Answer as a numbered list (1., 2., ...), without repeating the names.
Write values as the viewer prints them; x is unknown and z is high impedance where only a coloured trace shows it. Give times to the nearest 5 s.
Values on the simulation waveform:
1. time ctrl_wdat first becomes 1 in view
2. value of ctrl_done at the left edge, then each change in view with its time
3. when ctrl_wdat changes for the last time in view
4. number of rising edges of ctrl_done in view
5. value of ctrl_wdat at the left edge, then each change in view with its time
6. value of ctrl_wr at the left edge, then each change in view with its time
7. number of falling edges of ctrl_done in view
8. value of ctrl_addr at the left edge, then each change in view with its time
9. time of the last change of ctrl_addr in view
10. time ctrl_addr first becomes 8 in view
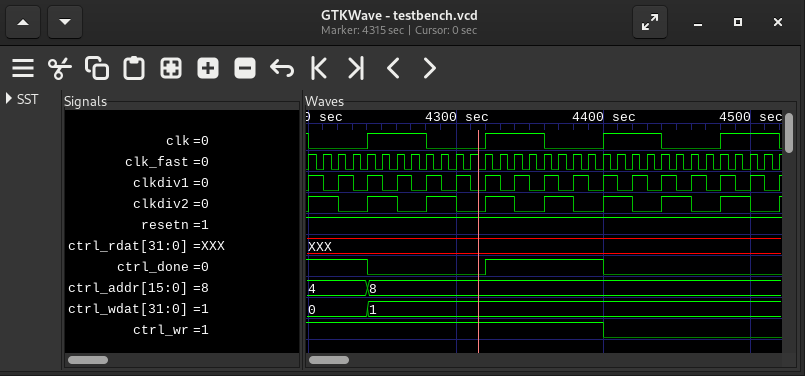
1. 4240 s
2. 1, 0 at 4240 s, 1 at 4320 s, 0 at 4400 s
3. 4240 s
4. 1
5. 0, 1 at 4240 s
6. 1, 0 at 4400 s
7. 2
8. 4, 8 at 4240 s
9. 4240 s
10. 4240 s
